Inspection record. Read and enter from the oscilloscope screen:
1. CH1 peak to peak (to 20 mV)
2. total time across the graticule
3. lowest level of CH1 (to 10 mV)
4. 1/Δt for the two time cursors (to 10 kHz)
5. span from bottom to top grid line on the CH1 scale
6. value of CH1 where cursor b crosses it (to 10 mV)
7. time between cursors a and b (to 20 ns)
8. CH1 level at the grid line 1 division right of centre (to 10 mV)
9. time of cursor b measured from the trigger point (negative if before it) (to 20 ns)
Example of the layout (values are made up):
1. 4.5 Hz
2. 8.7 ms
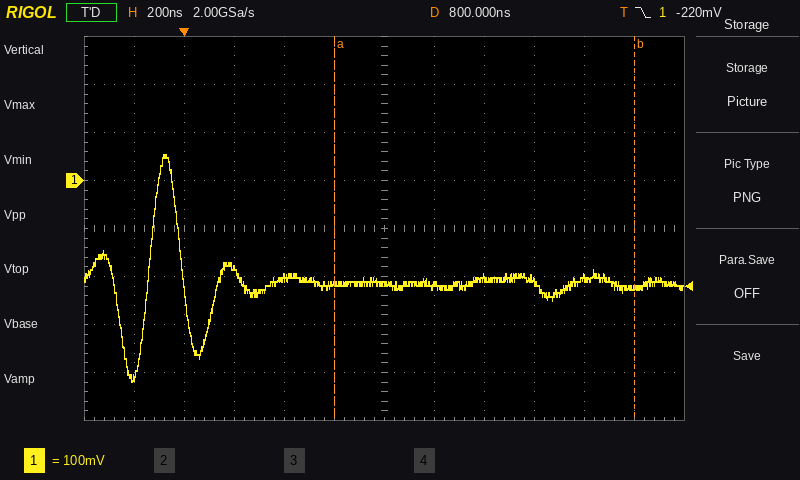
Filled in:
1. 480 mV
2. 2.4 µs
3. -420 mV
4. 830 kHz
5. 800 mV
6. -220 mV
7. 1.20 µs
8. -220 mV
9. +1.80 µs
